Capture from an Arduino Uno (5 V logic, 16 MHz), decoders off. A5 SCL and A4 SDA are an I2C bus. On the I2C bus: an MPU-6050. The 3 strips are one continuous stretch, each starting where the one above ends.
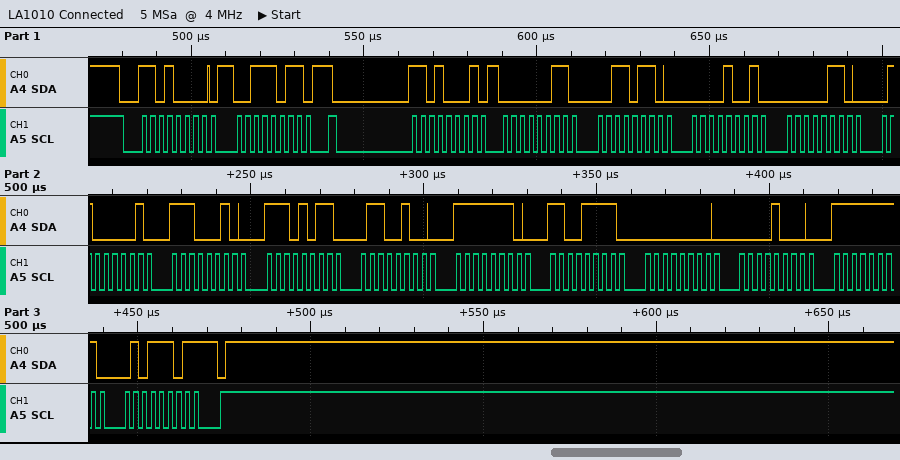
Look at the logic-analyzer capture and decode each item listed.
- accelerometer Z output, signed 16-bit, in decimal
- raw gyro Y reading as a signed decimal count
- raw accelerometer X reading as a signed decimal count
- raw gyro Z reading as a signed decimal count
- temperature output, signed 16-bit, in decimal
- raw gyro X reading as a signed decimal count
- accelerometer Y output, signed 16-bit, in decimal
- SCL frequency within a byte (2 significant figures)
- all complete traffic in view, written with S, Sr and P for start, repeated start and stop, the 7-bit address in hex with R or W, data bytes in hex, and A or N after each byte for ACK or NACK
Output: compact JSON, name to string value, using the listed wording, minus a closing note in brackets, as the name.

{"accelerometer Z output, signed 16-bit, in decimal": "16866", "raw gyro Y reading as a signed decimal count": "8", "raw accelerometer X reading as a signed decimal count": "822", "raw gyro Z reading as a signed decimal count": "-163", "temperature output, signed 16-bit, in decimal": "-5276", "raw gyro X reading as a signed decimal count": "-305", "accelerometer Y output, signed 16-bit, in decimal": "2310", "SCL frequency within a byte": "400 kHz", "all complete traffic in view, written with S, Sr and P for start, repeated start and stop, the 7-bit address in hex with R or W, data bytes in hex, and A or N after each byte for ACK or NACK": "S 68W A 3B A Sr 68R A 03 A 36 A 09 A 06 A 41 A E2 A EB A 64 A FE A CF A 00 A 08 A FF A 5D N P"}
